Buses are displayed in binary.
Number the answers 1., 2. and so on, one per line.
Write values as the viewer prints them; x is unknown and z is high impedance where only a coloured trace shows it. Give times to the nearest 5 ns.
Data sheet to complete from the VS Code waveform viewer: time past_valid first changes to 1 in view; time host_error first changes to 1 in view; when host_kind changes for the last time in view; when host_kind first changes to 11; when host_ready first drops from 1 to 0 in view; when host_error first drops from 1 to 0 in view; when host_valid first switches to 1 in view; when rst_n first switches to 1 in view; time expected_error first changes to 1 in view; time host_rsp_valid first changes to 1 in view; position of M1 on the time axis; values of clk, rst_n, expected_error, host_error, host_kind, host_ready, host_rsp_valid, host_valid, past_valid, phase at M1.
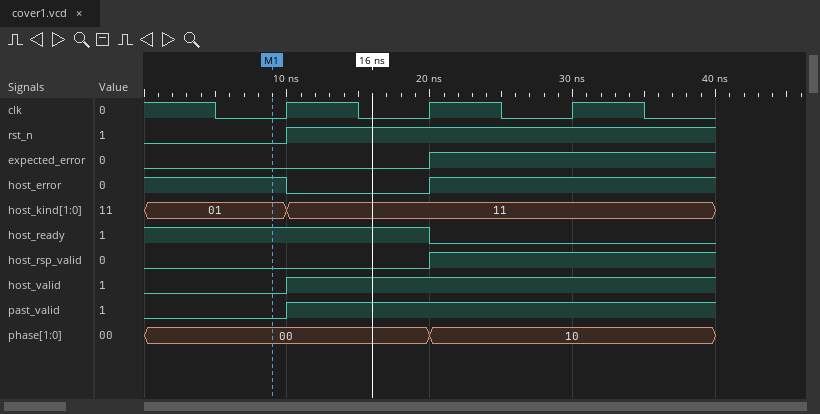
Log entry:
1. 10 ns
2. 20 ns
3. 10 ns
4. 10 ns
5. 20 ns
6. 10 ns
7. 10 ns
8. 10 ns
9. 20 ns
10. 20 ns
11. 10 ns
12. clk=0, rst_n=0, expected_error=0, host_error=1, host_kind=01, host_ready=1, host_rsp_valid=0, host_valid=0, past_valid=0, phase=00
